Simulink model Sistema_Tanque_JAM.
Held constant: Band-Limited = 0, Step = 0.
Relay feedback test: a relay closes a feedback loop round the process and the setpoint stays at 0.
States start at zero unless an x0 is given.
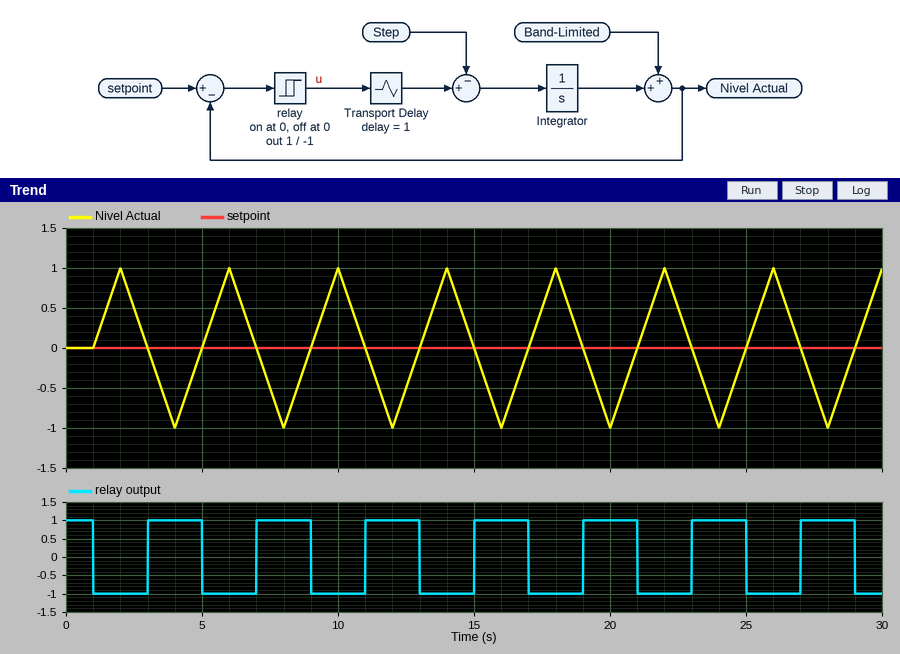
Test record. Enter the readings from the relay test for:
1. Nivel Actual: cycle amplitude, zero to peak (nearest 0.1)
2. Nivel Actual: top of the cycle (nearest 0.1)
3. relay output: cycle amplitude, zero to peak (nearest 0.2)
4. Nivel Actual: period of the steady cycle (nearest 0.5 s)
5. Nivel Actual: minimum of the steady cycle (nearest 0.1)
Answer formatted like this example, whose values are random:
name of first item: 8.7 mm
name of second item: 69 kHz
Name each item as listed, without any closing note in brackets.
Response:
Nivel Actual: cycle amplitude, zero to peak: 1.0
Nivel Actual: top of the cycle: 1.0
relay output: cycle amplitude, zero to peak: 1.0
Nivel Actual: period of the steady cycle: 4.0 s
Nivel Actual: minimum of the steady cycle: -1.0
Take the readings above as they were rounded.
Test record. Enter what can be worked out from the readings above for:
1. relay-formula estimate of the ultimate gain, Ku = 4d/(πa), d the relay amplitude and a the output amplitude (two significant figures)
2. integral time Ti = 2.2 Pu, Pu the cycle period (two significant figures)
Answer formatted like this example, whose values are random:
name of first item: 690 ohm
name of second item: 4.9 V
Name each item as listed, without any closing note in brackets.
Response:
relay-formula estimate of the ultimate gain, Ku = 4d/(πa), d the relay amplitude and a the output amplitude: 1.3
integral time Ti = 2.2 Pu, Pu the cycle period: 8.8 s
